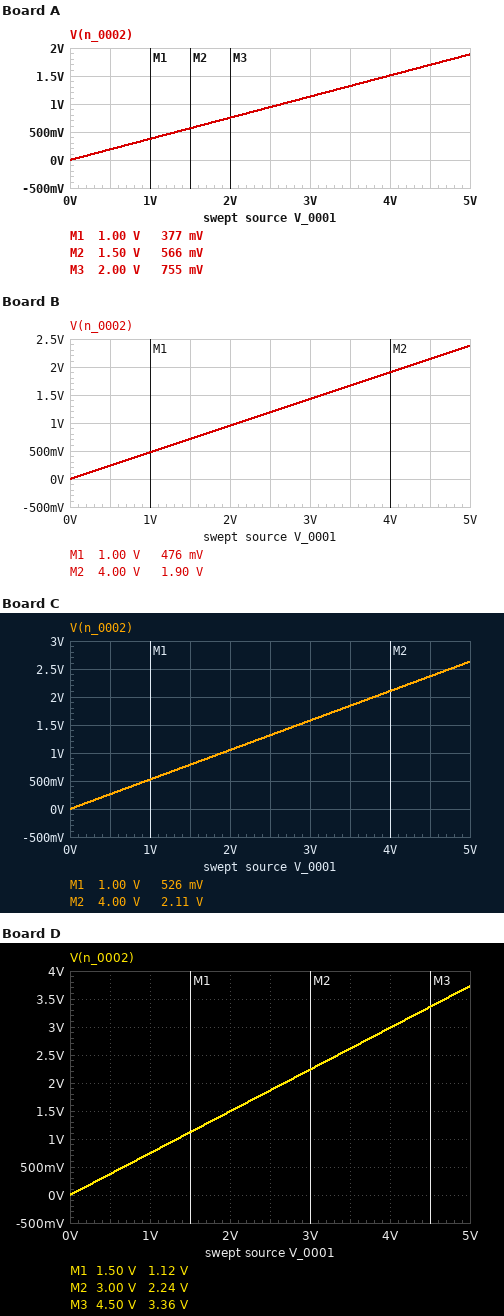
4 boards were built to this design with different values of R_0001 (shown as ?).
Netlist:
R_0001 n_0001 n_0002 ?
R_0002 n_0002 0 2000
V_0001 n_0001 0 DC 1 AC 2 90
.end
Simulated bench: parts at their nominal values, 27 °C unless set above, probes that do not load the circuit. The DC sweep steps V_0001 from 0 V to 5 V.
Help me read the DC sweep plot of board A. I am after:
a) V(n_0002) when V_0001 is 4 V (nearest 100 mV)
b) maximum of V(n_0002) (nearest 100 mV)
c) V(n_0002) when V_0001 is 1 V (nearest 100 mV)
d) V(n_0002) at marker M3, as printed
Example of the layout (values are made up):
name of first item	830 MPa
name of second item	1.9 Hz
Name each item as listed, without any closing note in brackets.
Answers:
V(n_0002) when V_0001 is 4 V	1.5 V
maximum of V(n_0002)	1.9 V
V(n_0002) when V_0001 is 1 V	400 mV
V(n_0002) at marker M3, as printed	755 mV
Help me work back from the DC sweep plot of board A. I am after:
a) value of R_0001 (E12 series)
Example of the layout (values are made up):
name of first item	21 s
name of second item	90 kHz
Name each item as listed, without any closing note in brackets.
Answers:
value of R_0001	3.3 kΩ
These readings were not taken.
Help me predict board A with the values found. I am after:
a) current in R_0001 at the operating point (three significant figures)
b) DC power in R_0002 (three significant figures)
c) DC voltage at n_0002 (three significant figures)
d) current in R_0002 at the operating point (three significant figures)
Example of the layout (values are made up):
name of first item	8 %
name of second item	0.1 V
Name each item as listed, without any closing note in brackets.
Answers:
current in R_0001 at the operating point	189 µA
DC power in R_0002	71.2 µW
DC voltage at n_0002	377 mV
current in R_0002 at the operating point	189 µA
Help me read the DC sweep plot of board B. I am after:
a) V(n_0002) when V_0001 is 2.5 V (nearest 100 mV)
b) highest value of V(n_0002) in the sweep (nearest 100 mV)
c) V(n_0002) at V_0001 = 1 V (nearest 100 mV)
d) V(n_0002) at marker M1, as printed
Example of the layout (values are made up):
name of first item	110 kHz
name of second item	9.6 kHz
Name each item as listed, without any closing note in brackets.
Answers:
V(n_0002) when V_0001 is 2.5 V	1.2 V
highest value of V(n_0002) in the sweep	2.4 V
V(n_0002) at V_0001 = 1 V	500 mV
V(n_0002) at marker M1, as printed	476 mV
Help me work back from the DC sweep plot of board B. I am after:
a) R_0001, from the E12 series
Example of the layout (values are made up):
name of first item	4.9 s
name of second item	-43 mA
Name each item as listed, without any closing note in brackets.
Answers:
R_0001, from the E12 series	2.2 kΩ
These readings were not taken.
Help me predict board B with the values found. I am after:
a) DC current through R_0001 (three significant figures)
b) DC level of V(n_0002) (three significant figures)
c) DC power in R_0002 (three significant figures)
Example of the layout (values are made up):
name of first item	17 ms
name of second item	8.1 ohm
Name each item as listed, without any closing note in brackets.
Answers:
DC current through R_0001	238 µA
DC level of V(n_0002)	476 mV
DC power in R_0002	113 µW
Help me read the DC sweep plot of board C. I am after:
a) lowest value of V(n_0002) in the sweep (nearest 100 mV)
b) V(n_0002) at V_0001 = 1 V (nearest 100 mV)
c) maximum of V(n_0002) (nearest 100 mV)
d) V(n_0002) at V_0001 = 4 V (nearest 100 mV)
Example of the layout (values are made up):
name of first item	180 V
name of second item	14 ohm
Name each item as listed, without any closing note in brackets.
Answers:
lowest value of V(n_0002) in the sweep	0 V
V(n_0002) at V_0001 = 1 V	500 mV
maximum of V(n_0002)	2.6 V
V(n_0002) at V_0001 = 4 V	2.1 V
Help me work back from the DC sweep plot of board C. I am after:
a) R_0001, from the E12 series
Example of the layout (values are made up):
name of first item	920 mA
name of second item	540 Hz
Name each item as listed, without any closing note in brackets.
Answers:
R_0001, from the E12 series	1.8 kΩ
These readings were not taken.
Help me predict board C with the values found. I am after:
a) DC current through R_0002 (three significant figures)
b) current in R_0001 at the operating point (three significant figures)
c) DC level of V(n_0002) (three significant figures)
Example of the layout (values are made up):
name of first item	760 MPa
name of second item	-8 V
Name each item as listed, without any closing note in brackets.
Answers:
DC current through R_0002	263 µA
current in R_0001 at the operating point	263 µA
DC level of V(n_0002)	526 mV
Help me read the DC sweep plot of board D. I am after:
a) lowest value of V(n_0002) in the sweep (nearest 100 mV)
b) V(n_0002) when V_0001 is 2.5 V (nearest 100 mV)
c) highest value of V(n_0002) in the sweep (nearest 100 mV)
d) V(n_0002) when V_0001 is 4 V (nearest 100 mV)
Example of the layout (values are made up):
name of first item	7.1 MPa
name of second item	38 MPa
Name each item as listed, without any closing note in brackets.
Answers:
lowest value of V(n_0002) in the sweep	0 V
V(n_0002) when V_0001 is 2.5 V	1.9 V
highest value of V(n_0002) in the sweep	3.7 V
V(n_0002) when V_0001 is 4 V	3.0 V
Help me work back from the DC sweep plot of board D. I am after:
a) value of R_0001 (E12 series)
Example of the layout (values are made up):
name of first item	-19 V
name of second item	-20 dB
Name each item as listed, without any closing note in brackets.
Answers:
value of R_0001	680 Ω
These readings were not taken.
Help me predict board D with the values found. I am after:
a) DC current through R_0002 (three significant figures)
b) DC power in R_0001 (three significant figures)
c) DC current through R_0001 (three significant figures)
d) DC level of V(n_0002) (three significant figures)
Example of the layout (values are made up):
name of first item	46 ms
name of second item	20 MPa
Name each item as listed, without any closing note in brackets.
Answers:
DC current through R_0002	373 µA
DC power in R_0001	94.7 µW
DC current through R_0001	373 µA
DC level of V(n_0002)	746 mV
